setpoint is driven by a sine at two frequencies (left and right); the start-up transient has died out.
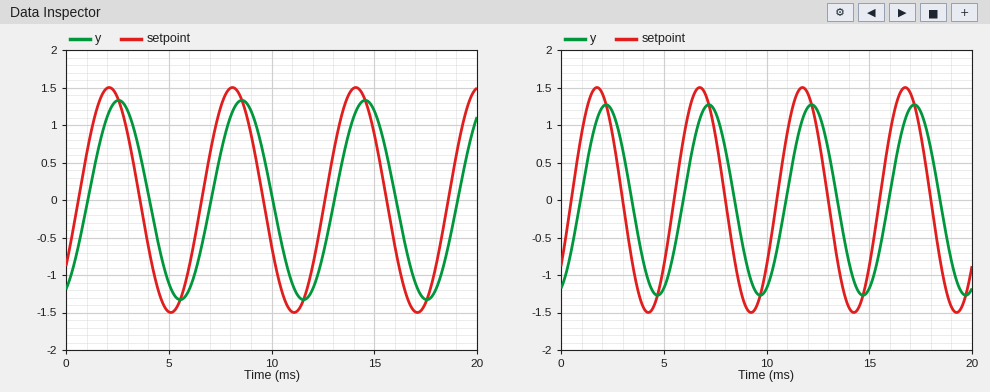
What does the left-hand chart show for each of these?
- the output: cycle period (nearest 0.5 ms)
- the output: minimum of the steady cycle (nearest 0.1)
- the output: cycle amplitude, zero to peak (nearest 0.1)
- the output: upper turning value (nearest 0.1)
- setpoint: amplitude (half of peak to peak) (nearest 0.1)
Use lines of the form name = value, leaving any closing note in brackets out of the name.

the output: cycle period = 6.0 ms
the output: minimum of the steady cycle = -1.3
the output: cycle amplitude, zero to peak = 1.3
the output: upper turning value = 1.3
setpoint: amplitude (half of peak to peak) = 1.5
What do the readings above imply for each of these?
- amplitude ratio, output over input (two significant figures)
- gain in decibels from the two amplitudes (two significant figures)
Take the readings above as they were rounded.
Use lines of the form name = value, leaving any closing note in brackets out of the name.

amplitude ratio, output over input = 0.87
gain in decibels from the two amplitudes = -1.2 dB
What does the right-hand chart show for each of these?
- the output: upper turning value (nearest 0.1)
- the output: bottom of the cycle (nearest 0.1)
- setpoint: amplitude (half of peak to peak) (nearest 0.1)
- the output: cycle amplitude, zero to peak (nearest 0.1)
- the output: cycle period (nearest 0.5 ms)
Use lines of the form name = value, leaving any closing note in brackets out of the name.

the output: upper turning value = 1.3
the output: bottom of the cycle = -1.3
setpoint: amplitude (half of peak to peak) = 1.5
the output: cycle amplitude, zero to peak = 1.3
the output: cycle period = 5.0 ms
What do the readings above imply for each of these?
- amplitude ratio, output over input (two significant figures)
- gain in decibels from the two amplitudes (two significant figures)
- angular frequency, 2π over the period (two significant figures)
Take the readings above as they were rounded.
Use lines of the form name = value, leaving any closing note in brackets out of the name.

amplitude ratio, output over input = 0.87
gain in decibels from the two amplitudes = -1.2 dB
angular frequency, 2π over the period = 1.3 rad/ms
